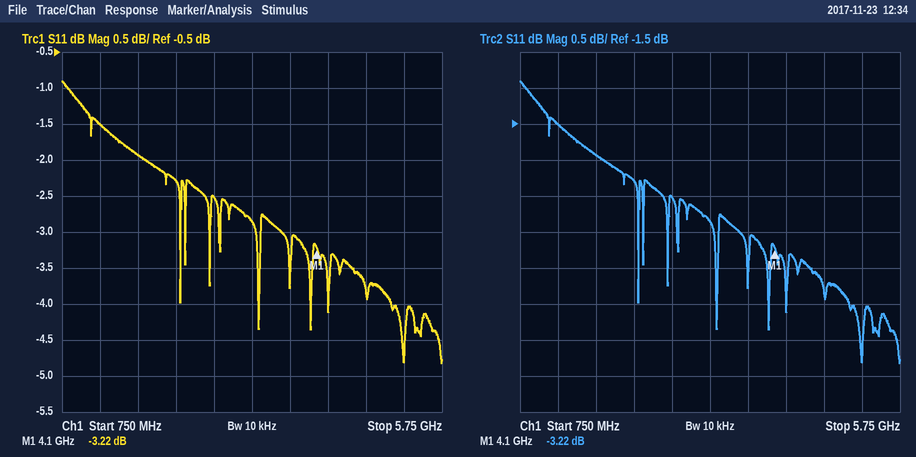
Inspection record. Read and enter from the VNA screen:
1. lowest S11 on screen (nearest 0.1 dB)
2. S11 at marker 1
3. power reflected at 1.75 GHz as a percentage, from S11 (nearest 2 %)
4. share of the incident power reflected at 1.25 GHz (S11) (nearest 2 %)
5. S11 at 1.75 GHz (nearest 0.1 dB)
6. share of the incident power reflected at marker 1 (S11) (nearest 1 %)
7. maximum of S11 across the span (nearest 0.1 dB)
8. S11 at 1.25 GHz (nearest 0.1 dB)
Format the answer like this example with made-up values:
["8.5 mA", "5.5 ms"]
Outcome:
["-4.8 dB", "-3.22 dB", "64 %", "70 %", "-1.9 dB", "48 %", "-0.9 dB", "-1.5 dB"]
